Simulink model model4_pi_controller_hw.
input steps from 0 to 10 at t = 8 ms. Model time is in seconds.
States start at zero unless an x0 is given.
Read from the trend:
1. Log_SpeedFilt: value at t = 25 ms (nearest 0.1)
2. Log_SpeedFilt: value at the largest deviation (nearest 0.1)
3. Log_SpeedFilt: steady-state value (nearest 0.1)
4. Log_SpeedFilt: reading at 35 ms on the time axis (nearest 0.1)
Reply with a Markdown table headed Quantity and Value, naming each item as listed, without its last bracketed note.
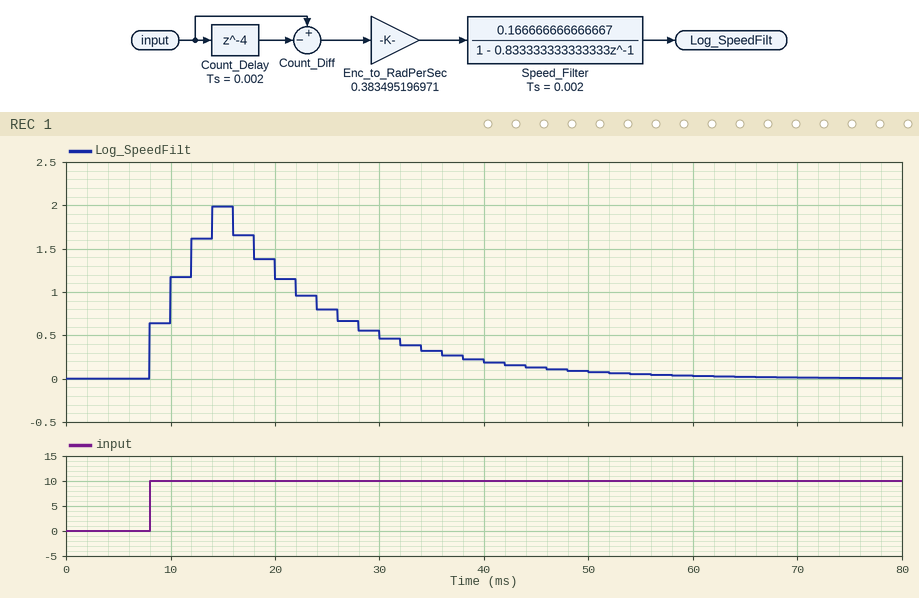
| Quantity | Value |
|---|---|
| Log_SpeedFilt: value at t = 25 ms | 0.8 |
| Log_SpeedFilt: value at the largest deviation | 2.0 |
| Log_SpeedFilt: steady-state value | 0.0 |
| Log_SpeedFilt: reading at 35 ms on the time axis | 0.3 |
